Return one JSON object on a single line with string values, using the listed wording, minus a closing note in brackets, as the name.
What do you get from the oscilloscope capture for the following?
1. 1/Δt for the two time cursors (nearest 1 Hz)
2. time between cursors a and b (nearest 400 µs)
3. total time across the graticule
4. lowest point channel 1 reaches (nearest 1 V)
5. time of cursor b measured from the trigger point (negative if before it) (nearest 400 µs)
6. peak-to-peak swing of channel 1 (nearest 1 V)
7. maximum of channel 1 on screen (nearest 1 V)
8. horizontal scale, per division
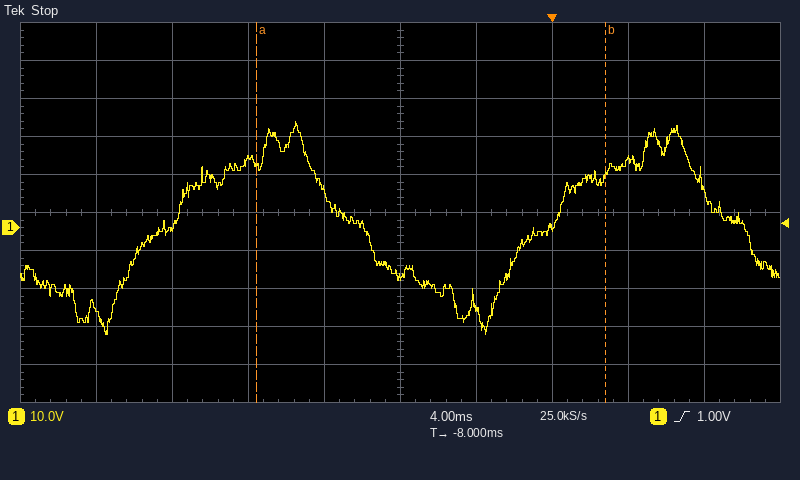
{"1/Δt for the two time cursors": "54 Hz", "time between cursors a and b": "18.4 ms", "total time across the graticule": "40 ms", "lowest point channel 1 reaches": "-28 V", "time of cursor b measured from the trigger point (negative if before it)": "+2.8 ms", "peak-to-peak swing of channel 1": "56 V", "maximum of channel 1 on screen": "28 V", "horizontal scale, per division": "4 ms"}
